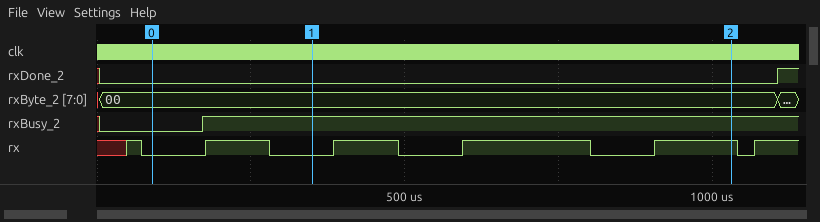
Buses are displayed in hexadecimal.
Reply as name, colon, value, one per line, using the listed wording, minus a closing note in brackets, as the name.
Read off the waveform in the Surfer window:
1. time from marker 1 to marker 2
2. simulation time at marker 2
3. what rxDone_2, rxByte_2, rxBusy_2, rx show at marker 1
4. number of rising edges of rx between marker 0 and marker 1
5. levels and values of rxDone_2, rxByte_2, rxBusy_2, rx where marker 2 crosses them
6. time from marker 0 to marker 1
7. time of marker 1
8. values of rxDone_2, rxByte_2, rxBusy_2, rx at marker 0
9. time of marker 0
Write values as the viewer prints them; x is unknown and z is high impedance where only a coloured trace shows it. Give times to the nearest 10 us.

time from marker 1 to marker 2: 680 us
simulation time at marker 2: 1030 us
what rxDone_2, rxByte_2, rxBusy_2, rx show at marker 1: rxDone_2=0, rxByte_2=00, rxBusy_2=1, rx=0
number of rising edges of rx between marker 0 and marker 1: 1
levels and values of rxDone_2, rxByte_2, rxBusy_2, rx where marker 2 crosses them: rxDone_2=0, rxByte_2=00, rxBusy_2=1, rx=1
time from marker 0 to marker 1: 260 us
time of marker 1: 350 us
values of rxDone_2, rxByte_2, rxBusy_2, rx at marker 0: rxDone_2=0, rxByte_2=00, rxBusy_2=0, rx=0
time of marker 0: 90 us
